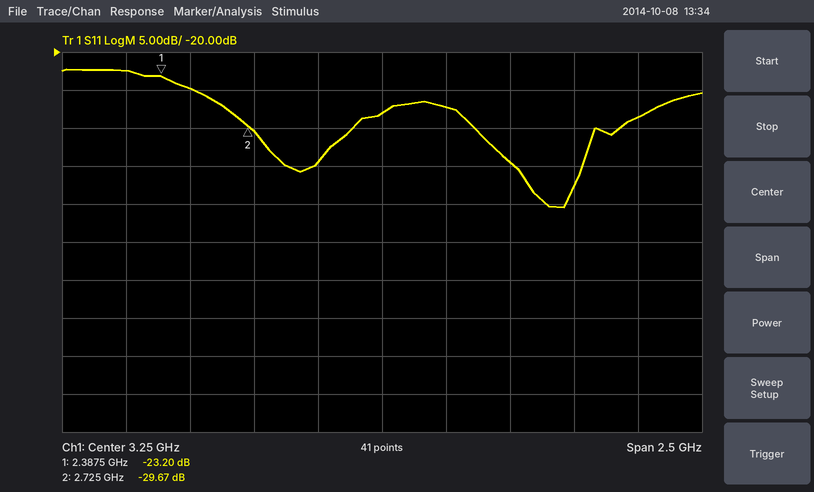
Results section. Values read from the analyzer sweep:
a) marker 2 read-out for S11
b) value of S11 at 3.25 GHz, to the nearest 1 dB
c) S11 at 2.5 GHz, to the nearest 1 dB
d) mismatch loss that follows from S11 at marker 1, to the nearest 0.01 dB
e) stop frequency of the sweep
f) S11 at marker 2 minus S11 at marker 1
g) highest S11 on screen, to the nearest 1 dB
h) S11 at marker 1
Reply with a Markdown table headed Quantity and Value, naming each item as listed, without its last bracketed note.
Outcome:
| Quantity | Value |
|---|---|
| marker 2 read-out for S11 | -29.67 dB |
| value of S11 at 3.25 GHz, to the nearest 1 dB | -28 dB |
| S11 at 2.5 GHz, to the nearest 1 dB | -25 dB |
| mismatch loss that follows from S11 at marker 1, to the nearest 0.01 dB | 0.02 dB |
| stop frequency of the sweep | 4.5 GHz |
| S11 at marker 2 minus S11 at marker 1 | -6.47 dB |
| highest S11 on screen, to the nearest 1 dB | -22 dB |
| S11 at marker 1 | -23.20 dB |
